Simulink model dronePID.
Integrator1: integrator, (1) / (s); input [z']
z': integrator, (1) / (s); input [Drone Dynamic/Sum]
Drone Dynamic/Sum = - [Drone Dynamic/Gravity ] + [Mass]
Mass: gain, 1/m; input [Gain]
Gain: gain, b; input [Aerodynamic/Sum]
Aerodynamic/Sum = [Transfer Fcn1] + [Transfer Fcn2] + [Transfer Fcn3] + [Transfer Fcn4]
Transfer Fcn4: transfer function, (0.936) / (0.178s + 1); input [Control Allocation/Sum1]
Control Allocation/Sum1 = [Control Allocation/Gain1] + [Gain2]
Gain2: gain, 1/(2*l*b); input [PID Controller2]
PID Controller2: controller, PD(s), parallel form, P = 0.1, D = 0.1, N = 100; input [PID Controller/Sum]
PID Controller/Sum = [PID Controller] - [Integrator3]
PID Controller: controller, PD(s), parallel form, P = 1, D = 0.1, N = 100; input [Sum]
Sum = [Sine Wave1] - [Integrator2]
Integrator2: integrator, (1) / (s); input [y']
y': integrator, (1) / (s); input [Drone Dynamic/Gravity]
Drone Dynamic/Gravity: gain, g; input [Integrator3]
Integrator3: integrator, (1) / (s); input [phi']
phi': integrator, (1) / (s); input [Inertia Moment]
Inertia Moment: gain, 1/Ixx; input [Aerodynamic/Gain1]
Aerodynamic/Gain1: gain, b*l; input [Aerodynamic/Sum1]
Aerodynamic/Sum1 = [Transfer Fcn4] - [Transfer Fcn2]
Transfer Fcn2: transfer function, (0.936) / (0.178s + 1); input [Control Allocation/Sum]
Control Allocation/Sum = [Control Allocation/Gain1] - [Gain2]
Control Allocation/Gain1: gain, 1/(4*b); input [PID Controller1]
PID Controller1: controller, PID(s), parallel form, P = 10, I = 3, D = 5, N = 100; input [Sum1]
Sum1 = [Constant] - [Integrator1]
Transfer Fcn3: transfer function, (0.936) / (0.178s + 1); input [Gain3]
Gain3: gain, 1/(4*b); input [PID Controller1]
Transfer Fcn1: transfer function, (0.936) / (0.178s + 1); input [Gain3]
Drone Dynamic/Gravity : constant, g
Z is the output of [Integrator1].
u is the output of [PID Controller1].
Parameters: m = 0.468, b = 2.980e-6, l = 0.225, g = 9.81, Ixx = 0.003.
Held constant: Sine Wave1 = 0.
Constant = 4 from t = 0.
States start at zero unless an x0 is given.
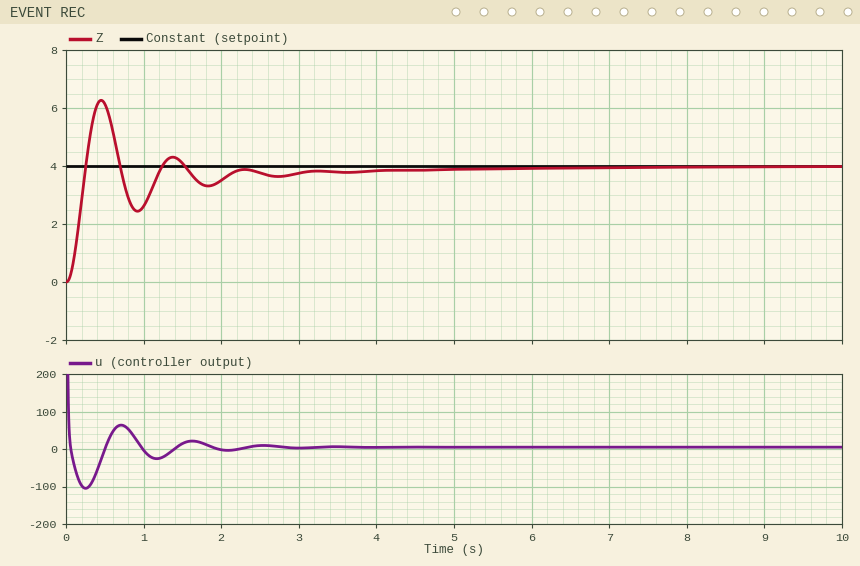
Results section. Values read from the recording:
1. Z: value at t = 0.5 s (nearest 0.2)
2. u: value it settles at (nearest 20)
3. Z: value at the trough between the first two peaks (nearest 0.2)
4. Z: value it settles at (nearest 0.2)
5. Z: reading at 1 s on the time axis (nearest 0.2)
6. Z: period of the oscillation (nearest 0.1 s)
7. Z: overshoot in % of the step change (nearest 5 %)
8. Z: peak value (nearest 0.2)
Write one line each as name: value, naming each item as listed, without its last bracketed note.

Z: value at t = 0.5 s: 6.2
u: value it settles at: 0
Z: value at the trough between the first two peaks: 2.4
Z: value it settles at: 4.0
Z: reading at 1 s on the time axis: 2.6
Z: period of the oscillation: 0.9 s
Z: overshoot in % of the step change: 55 %
Z: peak value: 6.2
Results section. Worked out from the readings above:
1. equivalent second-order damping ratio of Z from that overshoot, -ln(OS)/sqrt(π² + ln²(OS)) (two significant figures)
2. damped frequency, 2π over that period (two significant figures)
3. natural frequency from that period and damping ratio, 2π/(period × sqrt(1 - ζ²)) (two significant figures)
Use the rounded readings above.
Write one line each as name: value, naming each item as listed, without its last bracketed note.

equivalent second-order damping ratio of Z from that overshoot, -ln(OS)/sqrt(π² + ln²(OS)): 0.19
damped frequency, 2π over that period: 7.0 rad/s
natural frequency from that period and damping ratio, 2π/(period × sqrt(1 - ζ²)): 7.1 rad/s
